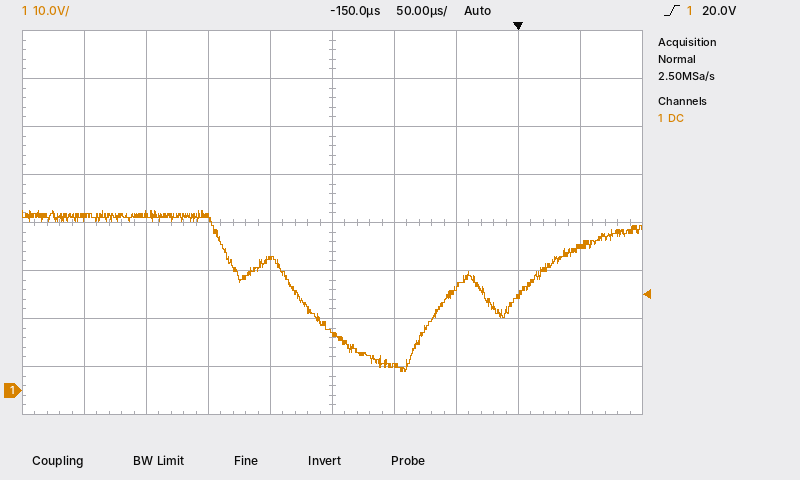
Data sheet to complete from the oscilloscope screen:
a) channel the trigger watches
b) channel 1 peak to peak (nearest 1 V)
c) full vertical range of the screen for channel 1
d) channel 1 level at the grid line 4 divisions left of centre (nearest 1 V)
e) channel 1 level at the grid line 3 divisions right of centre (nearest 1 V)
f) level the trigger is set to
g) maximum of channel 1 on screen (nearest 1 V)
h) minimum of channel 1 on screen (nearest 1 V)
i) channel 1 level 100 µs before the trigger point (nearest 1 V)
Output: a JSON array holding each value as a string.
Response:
["channel 1", "34 V", "80 V", "36 V", "20 V", "20.0 V", "38 V", "4 V", "5 V"]
